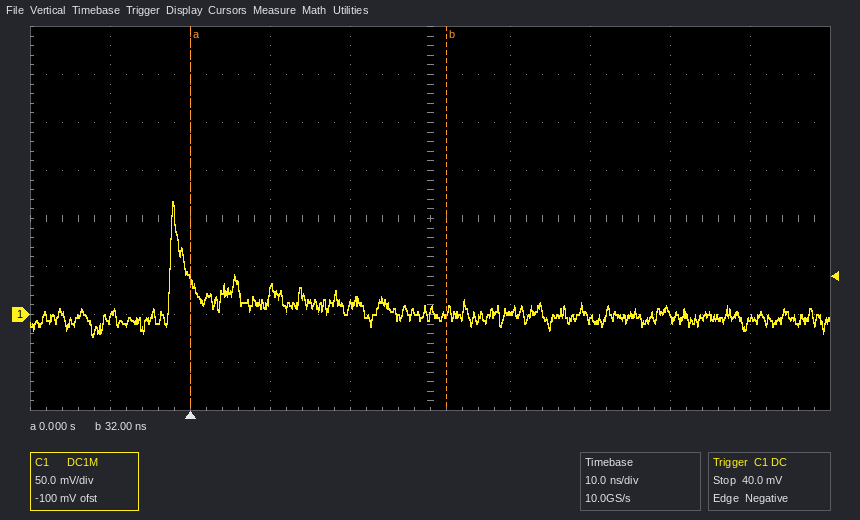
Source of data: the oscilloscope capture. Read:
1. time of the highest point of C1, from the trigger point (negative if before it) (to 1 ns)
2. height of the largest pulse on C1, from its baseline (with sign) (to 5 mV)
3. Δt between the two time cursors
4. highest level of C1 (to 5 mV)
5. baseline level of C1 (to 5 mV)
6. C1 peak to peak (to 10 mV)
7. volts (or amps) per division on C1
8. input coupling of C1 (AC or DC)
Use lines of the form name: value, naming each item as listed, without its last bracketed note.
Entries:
time of the highest point of C1, from the trigger point (negative if before it): -2 ns
height of the largest pulse on C1, from its baseline (with sign): +120 mV
Δt between the two time cursors: 32 ns
highest level of C1: 120 mV
baseline level of C1: 0 mV
C1 peak to peak: 140 mV
volts (or amps) per division on C1: 50 mV
input coupling of C1: DC
